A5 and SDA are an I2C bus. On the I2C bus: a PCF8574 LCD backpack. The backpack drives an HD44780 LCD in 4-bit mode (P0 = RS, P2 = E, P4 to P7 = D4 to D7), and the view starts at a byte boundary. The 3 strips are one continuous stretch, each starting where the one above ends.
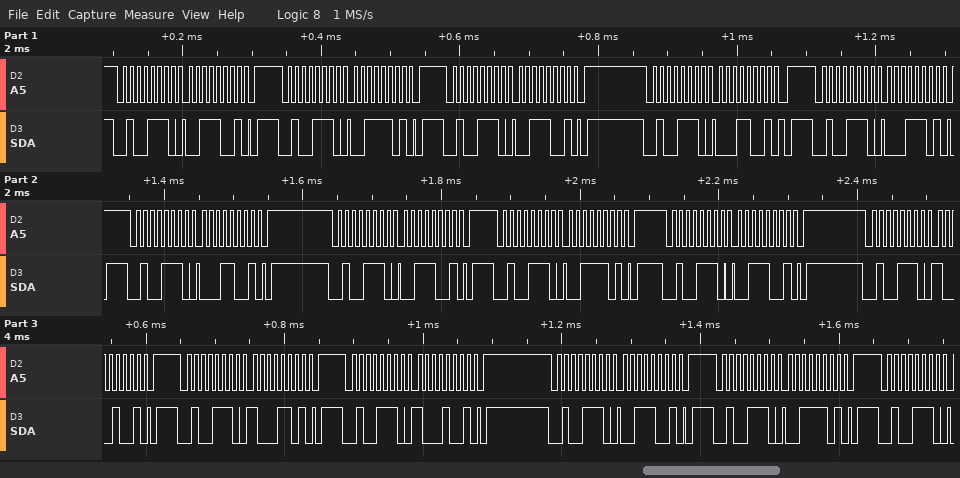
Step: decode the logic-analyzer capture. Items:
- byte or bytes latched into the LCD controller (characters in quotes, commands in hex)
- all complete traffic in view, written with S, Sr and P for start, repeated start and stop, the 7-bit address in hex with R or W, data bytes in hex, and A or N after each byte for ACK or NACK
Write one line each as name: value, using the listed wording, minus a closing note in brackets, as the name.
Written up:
byte or bytes latched into the LCD controller: '1' '8'
all complete traffic in view, written with S, Sr and P for start, repeated start and stop, the 7-bit address in hex with R or W, data bytes in hex, and A or N after each byte for ACK or NACK: S 27W A 39 A P S 27W A 3D A P S 27W A 39 A P S 27W A 19 A P S 27W A 1D A P S 27W A 19 A P S 27W A 39 A P S 27W A 3D A P S 27W A 39 A P S 27W A 89 A P S 27W A 8D A P S 27W A 89 A P S 27W A 39 A P S 27W A 3D A P S 27W A
